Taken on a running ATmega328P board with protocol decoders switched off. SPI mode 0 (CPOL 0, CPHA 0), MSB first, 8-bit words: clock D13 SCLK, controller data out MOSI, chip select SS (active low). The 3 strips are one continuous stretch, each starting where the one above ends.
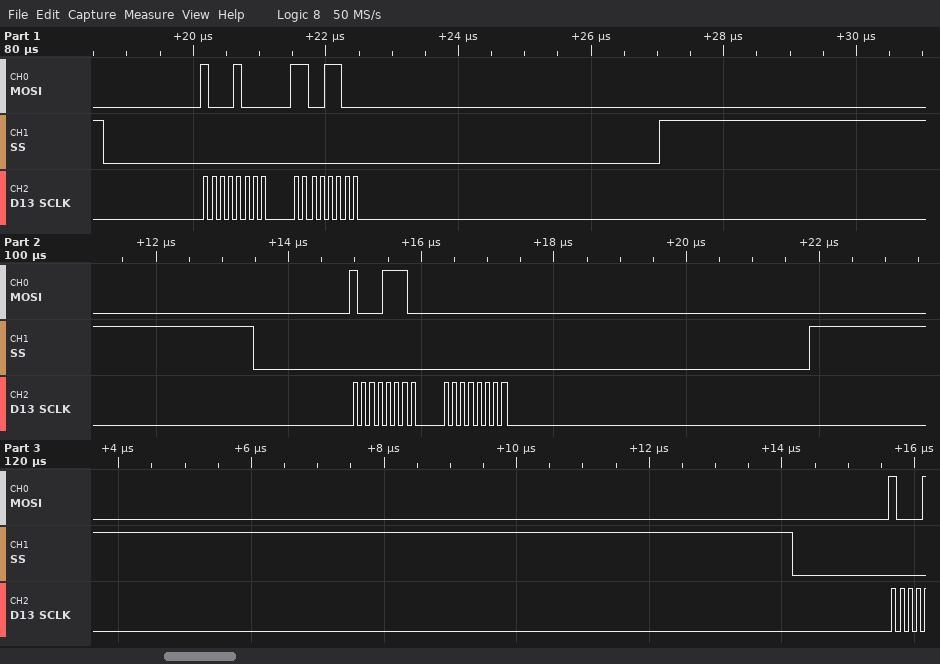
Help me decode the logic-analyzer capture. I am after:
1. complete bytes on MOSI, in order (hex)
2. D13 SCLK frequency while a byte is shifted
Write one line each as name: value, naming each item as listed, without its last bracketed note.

complete bytes on MOSI, in order: 0x88 0xCC 0x8E 0x00
D13 SCLK frequency while a byte is shifted: 8 MHz
